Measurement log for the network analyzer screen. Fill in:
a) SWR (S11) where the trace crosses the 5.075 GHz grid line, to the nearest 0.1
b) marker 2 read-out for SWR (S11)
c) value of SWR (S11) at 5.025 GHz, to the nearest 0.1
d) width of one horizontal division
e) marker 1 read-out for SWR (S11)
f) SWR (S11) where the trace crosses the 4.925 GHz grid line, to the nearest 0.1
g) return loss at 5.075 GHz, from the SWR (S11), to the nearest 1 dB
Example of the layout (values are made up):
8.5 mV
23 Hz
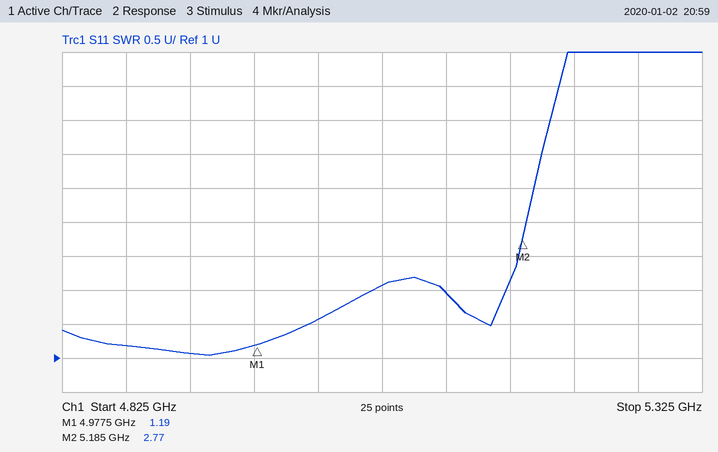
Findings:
2.1
2.77
1.6
50 MHz
1.19
1.1
9 dB
